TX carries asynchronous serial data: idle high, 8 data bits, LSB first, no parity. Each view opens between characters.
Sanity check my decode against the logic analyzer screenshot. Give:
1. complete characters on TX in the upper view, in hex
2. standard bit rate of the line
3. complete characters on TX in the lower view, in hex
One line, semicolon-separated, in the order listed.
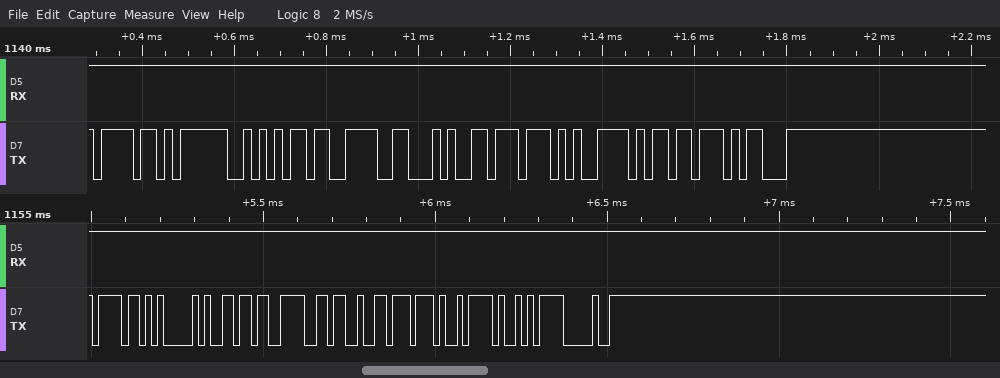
6F, 3F, B5, 9E, 94, 77, 79, DB, 8D; 57600 baud; 6F, 41, B6, 9E, 93, 77, 7A, EA, 90
